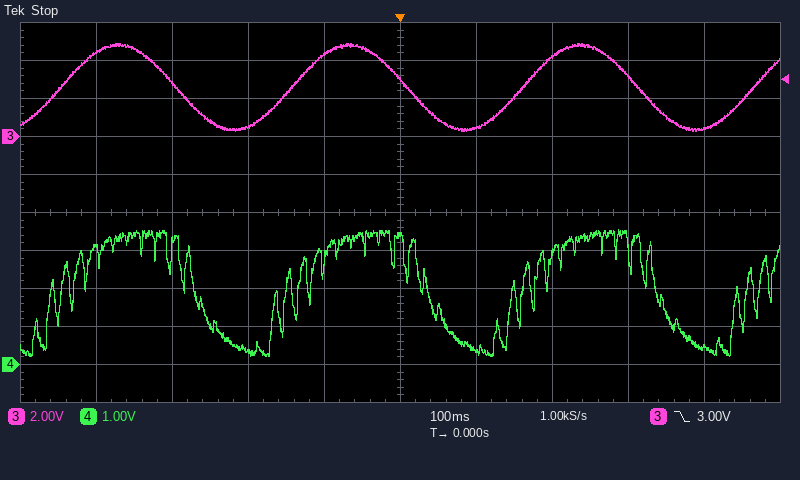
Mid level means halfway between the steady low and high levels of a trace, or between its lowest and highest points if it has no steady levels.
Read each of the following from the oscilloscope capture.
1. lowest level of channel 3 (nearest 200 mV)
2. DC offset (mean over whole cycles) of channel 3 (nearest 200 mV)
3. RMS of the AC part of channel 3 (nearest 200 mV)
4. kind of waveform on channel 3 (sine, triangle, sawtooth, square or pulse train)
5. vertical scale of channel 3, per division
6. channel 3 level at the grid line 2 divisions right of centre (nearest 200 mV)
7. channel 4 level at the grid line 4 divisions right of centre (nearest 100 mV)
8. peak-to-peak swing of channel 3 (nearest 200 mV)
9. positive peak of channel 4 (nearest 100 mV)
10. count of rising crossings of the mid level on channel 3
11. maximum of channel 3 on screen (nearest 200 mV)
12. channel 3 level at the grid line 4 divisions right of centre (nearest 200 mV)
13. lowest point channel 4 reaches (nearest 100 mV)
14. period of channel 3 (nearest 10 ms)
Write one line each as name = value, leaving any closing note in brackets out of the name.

lowest level of channel 3 = 200 mV
DC offset (mean over whole cycles) of channel 3 = 2.6 V
RMS of the AC part of channel 3 = 1.6 V
kind of waveform on channel 3 = sine
vertical scale of channel 3, per division = 2 V
channel 3 level at the grid line 2 divisions right of centre = 4.2 V
channel 4 level at the grid line 4 divisions right of centre = 400 mV
peak-to-peak swing of channel 3 = 4.6 V
positive peak of channel 4 = 3.6 V
count of rising crossings of the mid level on channel 3 = 4
maximum of channel 3 on screen = 4.8 V
channel 3 level at the grid line 4 divisions right of centre = 400 mV
lowest point channel 4 reaches = 200 mV
period of channel 3 = 300 ms
